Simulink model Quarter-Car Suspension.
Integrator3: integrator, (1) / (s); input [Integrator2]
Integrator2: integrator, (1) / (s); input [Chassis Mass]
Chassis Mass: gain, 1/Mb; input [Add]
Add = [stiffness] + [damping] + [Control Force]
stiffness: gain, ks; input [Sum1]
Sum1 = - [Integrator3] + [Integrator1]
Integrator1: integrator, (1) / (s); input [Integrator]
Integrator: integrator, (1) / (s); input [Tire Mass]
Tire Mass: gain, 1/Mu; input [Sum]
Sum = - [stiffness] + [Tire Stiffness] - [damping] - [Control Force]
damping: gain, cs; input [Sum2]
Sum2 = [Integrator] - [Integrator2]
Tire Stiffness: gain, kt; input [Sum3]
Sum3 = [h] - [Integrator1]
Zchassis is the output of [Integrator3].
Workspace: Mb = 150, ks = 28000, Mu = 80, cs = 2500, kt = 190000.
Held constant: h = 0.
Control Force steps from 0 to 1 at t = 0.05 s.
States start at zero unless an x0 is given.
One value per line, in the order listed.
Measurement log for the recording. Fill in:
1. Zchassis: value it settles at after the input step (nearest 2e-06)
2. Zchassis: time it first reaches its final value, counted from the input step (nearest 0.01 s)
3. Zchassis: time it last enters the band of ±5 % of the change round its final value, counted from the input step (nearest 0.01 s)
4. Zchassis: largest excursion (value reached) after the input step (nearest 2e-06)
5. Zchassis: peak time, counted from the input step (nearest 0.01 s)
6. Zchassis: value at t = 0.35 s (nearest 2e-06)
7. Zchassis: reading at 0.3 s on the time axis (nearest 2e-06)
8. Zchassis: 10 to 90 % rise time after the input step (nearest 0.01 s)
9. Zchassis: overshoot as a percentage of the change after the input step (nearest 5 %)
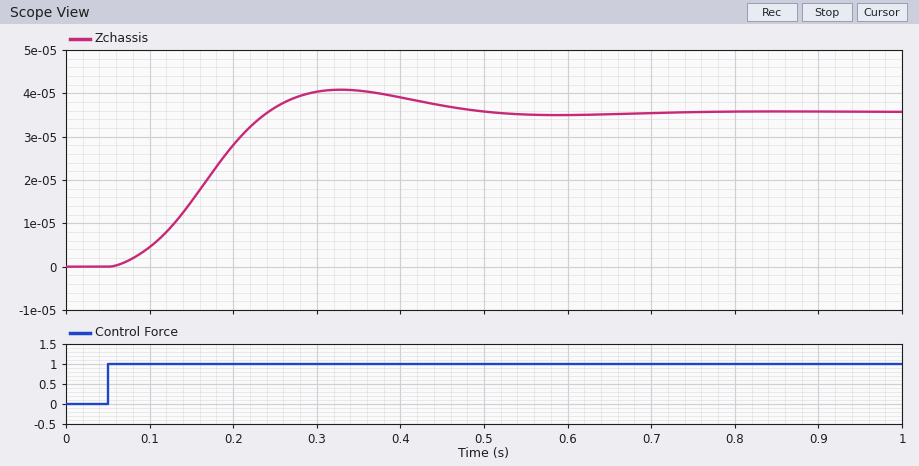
0.000036
0.19 s
0.39 s
0.000040
0.28 s
0.000040
0.000040
0.13 s
15 %
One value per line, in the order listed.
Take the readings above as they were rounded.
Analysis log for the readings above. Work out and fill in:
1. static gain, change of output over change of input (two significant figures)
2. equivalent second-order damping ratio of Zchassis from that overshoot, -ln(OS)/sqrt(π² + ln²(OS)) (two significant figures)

0.000036
0.52
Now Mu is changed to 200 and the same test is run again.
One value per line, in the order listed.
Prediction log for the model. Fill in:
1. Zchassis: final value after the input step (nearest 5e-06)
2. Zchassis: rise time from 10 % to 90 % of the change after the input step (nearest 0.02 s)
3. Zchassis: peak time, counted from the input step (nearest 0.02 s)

0.000035
0.14 s
0.26 s
